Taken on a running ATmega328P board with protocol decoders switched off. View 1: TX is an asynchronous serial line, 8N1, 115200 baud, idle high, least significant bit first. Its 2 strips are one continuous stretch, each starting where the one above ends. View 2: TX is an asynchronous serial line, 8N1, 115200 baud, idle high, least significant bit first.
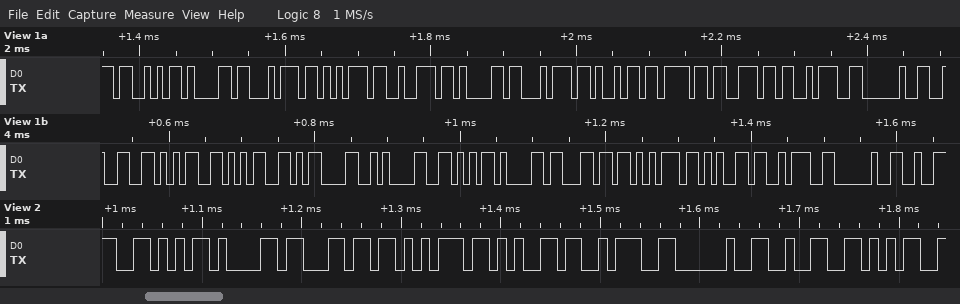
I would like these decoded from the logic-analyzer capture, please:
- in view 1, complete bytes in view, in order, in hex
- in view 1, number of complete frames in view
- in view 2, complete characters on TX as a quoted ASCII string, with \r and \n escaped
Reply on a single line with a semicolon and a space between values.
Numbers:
53 61 74 75 72 61 74 69 6F 6E 3A 20 32 35 35 0D 0A 56 61 6C 75 65 3A 20; 24; "Value: 25"
